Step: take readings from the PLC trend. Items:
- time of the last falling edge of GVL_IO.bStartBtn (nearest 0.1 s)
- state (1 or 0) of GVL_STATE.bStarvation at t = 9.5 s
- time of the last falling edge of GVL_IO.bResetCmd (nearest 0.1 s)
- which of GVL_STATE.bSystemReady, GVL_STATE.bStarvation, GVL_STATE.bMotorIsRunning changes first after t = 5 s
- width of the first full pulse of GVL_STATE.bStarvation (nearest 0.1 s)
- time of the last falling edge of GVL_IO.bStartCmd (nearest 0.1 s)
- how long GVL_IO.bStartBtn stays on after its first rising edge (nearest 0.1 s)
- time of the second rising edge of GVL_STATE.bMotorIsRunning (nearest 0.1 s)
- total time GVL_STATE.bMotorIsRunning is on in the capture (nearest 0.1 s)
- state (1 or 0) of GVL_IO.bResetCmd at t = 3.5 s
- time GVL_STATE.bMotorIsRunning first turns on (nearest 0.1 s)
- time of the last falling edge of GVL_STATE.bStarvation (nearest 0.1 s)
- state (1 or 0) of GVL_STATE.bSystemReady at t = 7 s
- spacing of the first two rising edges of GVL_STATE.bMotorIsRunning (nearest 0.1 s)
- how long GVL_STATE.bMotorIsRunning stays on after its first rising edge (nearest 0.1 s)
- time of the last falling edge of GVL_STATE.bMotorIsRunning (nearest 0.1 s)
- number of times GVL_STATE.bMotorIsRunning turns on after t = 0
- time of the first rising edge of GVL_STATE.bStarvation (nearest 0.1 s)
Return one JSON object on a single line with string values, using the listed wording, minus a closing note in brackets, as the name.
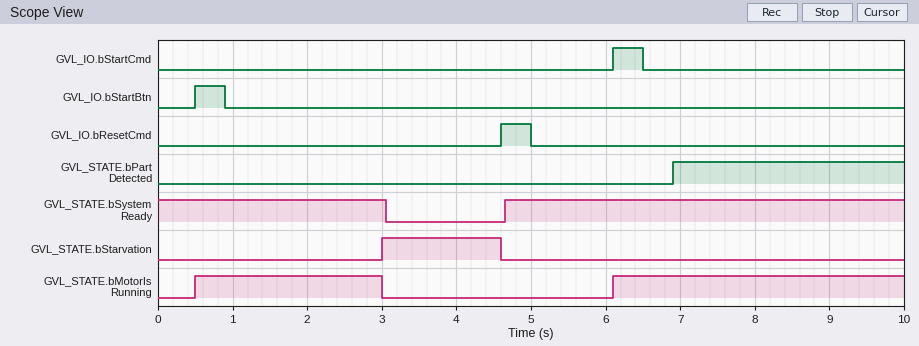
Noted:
{"time of the last falling edge of GVL_IO.bStartBtn": "0.9 s", "state (1 or 0) of GVL_STATE.bStarvation at t = 9.5 s": "0", "time of the last falling edge of GVL_IO.bResetCmd": "5.0 s", "which of GVL_STATE.bSystemReady, GVL_STATE.bStarvation, GVL_STATE.bMotorIsRunning changes first after t = 5 s": "GVL_STATE.bMotorIsRunning", "width of the first full pulse of GVL_STATE.bStarvation": "1.6 s", "time of the last falling edge of GVL_IO.bStartCmd": "6.5 s", "how long GVL_IO.bStartBtn stays on after its first rising edge": "0.4 s", "time of the second rising edge of GVL_STATE.bMotorIsRunning": "6.1 s", "total time GVL_STATE.bMotorIsRunning is on in the capture": "6.4 s", "state (1 or 0) of GVL_IO.bResetCmd at t = 3.5 s": "0", "time GVL_STATE.bMotorIsRunning first turns on": "0.5 s", "time of the last falling edge of GVL_STATE.bStarvation": "4.6 s", "state (1 or 0) of GVL_STATE.bSystemReady at t = 7 s": "1", "spacing of the first two rising edges of GVL_STATE.bMotorIsRunning": "5.6 s", "how long GVL_STATE.bMotorIsRunning stays on after its first rising edge": "2.5 s", "time of the last falling edge of GVL_STATE.bMotorIsRunning": "3.0 s", "number of times GVL_STATE.bMotorIsRunning turns on after t = 0": "2", "time of the first rising edge of GVL_STATE.bStarvation": "3.0 s"}
